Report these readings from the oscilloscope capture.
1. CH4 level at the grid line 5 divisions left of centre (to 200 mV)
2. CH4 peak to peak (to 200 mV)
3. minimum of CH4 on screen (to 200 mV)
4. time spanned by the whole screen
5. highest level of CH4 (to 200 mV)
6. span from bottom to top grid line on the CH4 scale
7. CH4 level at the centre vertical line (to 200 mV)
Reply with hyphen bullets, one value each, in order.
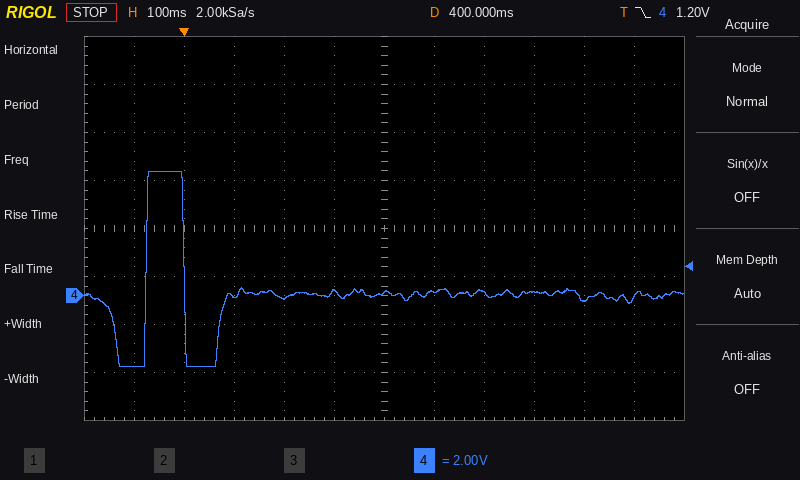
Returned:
- -3.0 V
- 8.2 V
- -3.0 V
- 1.2 s
- 5.2 V
- 16 V
- 200 mV
